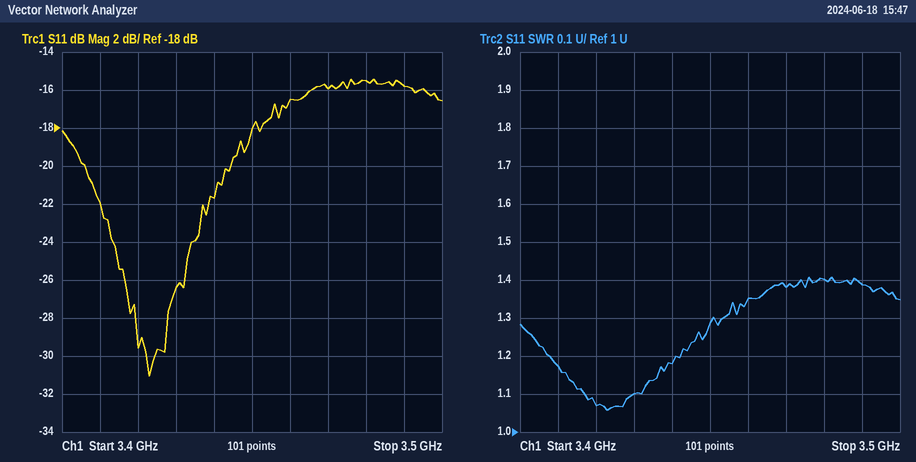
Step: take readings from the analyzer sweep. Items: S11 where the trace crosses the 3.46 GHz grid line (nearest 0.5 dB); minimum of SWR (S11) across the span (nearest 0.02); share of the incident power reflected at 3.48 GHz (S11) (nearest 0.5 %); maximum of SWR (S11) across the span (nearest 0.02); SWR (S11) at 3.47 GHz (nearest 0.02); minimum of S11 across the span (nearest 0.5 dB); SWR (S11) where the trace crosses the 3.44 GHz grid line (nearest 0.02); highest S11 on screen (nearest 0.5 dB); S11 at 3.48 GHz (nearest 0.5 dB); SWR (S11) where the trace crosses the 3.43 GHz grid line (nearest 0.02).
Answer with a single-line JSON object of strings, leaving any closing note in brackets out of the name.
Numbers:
{"S11 where the trace crosses the 3.46 GHz grid line": "-16.5 dB", "minimum of SWR (S11) across the span": "1.06", "share of the incident power reflected at 3.48 GHz (S11)": "3.0 %", "maximum of SWR (S11) across the span": "1.40", "SWR (S11) at 3.47 GHz": "1.38", "minimum of S11 across the span": "-31.0 dB", "SWR (S11) where the trace crosses the 3.44 GHz grid line": "1.18", "highest S11 on screen": "-15.5 dB", "S11 at 3.48 GHz": "-15.5 dB", "SWR (S11) where the trace crosses the 3.43 GHz grid line": "1.10"}
